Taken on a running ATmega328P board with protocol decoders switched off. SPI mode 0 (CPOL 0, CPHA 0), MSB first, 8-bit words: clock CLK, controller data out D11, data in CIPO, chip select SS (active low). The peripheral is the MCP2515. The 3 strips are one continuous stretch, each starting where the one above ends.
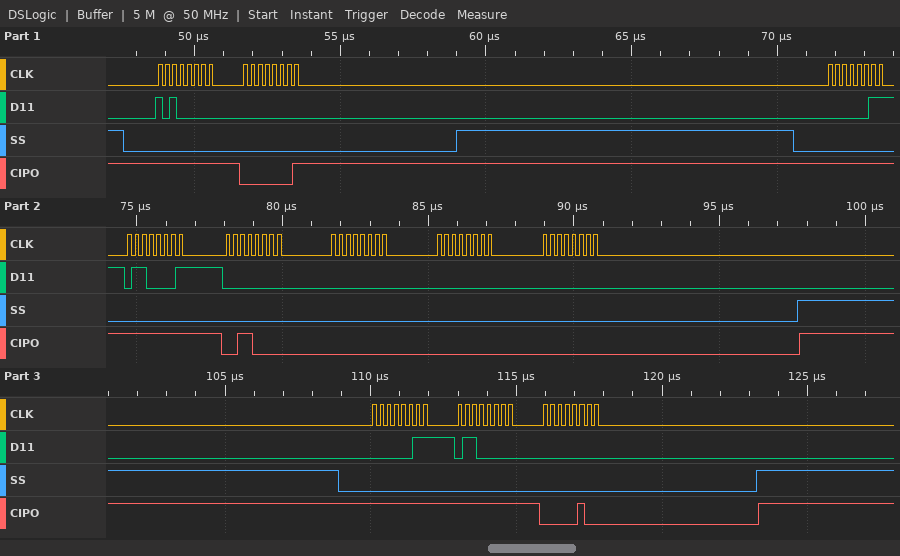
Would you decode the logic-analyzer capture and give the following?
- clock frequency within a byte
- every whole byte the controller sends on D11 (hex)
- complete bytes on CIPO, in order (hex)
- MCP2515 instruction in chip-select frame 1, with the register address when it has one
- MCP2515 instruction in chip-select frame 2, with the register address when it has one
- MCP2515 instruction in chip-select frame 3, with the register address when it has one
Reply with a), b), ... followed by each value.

a) 4 MHz
b) A0 00 03 61 00 00 00 00 03 60 00
c) FF 01 FF FF 30 00 00 00 FF FF 04
d) READ STATUS
e) READ 0x61
f) READ 0x60
